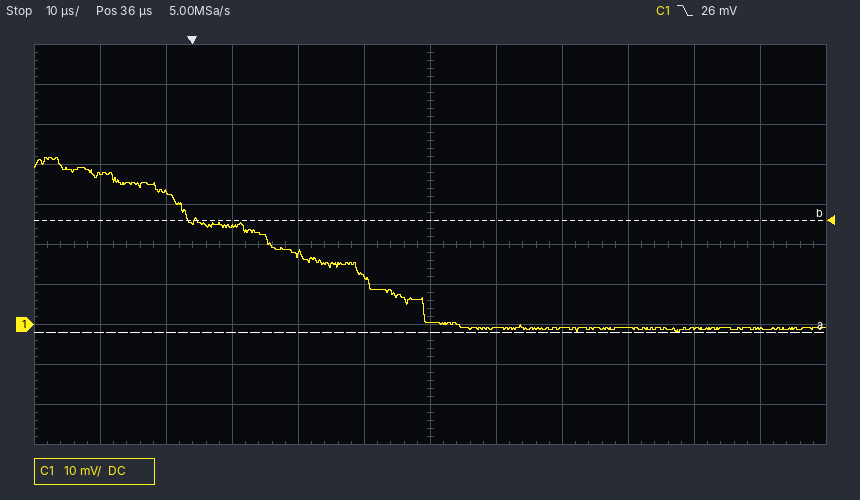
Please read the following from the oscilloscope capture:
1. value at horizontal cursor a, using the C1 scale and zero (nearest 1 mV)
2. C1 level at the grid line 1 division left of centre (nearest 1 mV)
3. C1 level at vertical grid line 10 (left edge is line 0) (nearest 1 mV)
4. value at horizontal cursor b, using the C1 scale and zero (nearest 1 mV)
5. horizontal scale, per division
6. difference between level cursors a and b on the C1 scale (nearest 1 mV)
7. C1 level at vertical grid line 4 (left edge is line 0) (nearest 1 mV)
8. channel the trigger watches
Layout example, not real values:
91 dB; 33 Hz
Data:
-2 mV; 12 mV; -1 mV; 26 mV; 10 µs; 28 mV; 18 mV; C1
